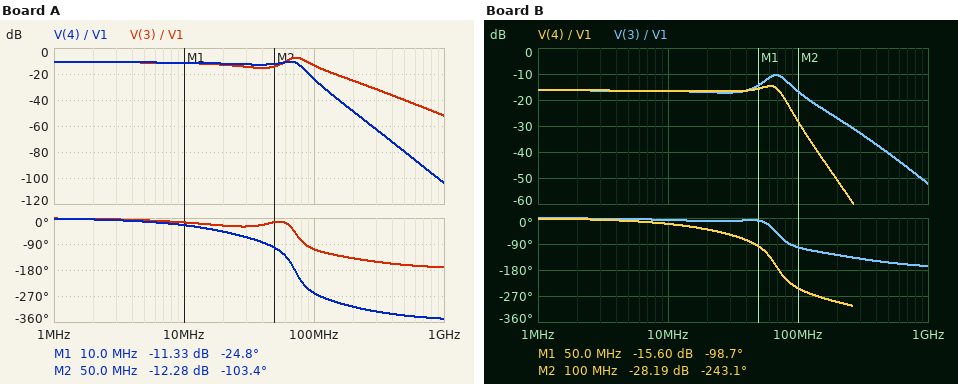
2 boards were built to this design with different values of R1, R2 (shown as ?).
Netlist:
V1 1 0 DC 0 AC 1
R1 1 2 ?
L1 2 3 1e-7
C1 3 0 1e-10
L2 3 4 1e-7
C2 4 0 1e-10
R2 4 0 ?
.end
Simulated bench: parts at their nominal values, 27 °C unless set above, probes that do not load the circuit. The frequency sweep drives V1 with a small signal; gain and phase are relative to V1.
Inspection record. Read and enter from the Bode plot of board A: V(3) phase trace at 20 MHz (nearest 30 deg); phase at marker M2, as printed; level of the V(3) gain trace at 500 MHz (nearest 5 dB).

-30 deg
-103.4 deg
-40 dB
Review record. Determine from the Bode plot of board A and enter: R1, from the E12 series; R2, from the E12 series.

100 Ω
39 Ω
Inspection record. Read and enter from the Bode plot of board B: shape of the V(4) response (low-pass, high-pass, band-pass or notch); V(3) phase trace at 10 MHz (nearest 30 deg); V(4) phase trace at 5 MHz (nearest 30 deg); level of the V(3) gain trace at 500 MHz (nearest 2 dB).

low-pass
0 deg
0 deg
-40 dB
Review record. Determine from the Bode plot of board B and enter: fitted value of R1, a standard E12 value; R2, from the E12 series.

150 Ω
27 Ω
